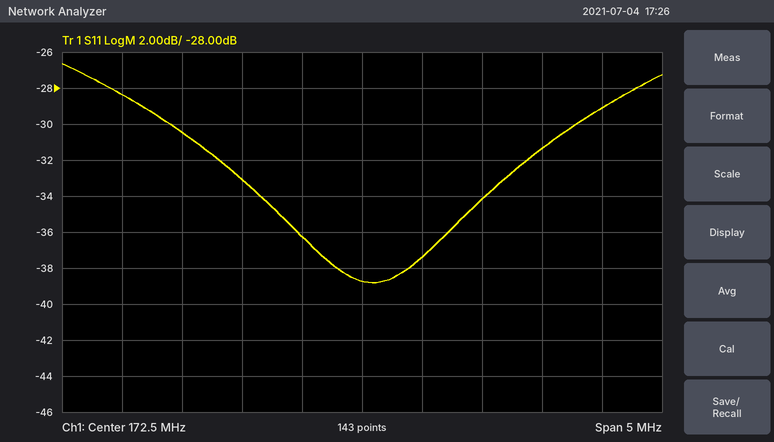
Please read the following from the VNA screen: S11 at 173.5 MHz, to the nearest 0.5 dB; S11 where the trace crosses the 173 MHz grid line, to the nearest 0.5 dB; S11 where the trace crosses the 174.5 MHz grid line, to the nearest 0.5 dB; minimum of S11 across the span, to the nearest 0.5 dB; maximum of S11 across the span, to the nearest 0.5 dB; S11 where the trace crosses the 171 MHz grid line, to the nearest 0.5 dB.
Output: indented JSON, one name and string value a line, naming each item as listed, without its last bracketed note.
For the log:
{
  "S11 at 173.5 MHz, to the nearest 0.5 dB": "-34.0 dB",
  "S11 where the trace crosses the 173 MHz grid line, to the nearest 0.5 dB": "-37.5 dB",
  "S11 where the trace crosses the 174.5 MHz grid line, to the nearest 0.5 dB": "-29.0 dB",
  "minimum of S11 across the span, to the nearest 0.5 dB": "-39.0 dB",
  "maximum of S11 across the span, to the nearest 0.5 dB": "-26.5 dB",
  "S11 where the trace crosses the 171 MHz grid line, to the nearest 0.5 dB": "-30.5 dB"
}
